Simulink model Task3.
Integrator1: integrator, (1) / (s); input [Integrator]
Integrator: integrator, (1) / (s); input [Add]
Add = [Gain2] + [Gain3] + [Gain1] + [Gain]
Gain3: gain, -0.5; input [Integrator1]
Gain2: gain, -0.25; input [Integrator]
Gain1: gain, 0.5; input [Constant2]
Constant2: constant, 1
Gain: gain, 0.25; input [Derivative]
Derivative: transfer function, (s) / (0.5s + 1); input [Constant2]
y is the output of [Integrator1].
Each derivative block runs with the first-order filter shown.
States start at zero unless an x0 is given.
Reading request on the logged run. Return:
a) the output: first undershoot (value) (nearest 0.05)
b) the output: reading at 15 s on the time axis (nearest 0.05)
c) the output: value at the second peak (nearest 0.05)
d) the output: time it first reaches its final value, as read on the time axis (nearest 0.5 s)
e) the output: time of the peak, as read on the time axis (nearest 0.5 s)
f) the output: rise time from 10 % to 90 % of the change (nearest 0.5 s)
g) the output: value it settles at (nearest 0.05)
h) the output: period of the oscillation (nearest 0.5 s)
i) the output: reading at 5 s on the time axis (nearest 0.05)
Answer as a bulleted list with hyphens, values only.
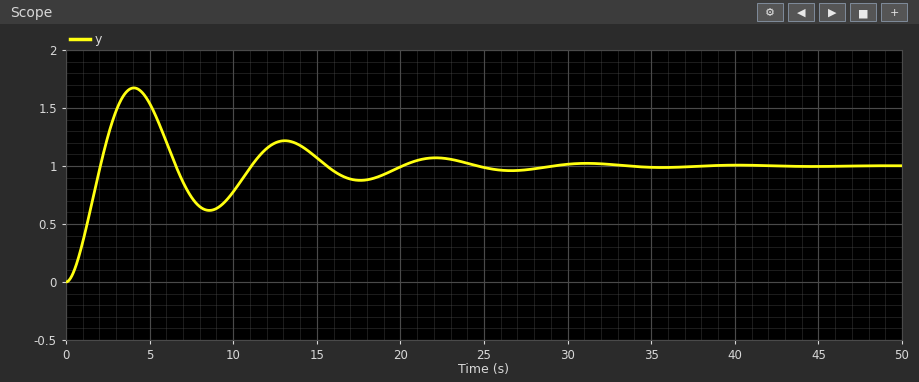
- 0.60
- 1.05
- 1.20
- 2.0 s
- 4.0 s
- 1.5 s
- 1.00
- 9.0 s
- 1.55
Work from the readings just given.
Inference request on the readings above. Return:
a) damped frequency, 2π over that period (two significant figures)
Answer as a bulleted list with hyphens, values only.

- 0.70 rad/s
